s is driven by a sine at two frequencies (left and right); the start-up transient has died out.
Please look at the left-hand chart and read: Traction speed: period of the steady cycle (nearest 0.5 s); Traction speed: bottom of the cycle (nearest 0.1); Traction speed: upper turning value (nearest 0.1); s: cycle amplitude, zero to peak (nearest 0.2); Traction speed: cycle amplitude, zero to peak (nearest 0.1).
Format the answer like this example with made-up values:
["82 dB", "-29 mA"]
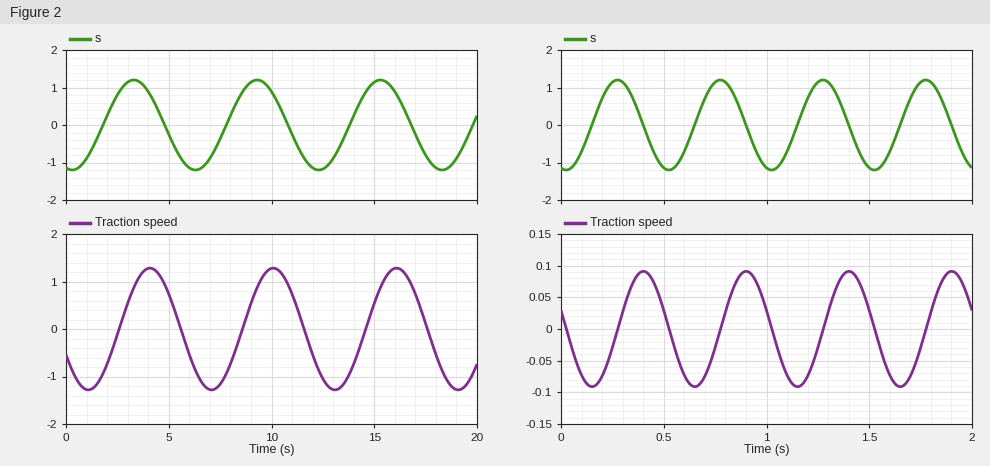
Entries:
["6.0 s", "-1.3", "1.3", "1.2", "1.3"]
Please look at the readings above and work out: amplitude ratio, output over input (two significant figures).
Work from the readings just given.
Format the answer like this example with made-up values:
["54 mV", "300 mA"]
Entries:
["1.1"]
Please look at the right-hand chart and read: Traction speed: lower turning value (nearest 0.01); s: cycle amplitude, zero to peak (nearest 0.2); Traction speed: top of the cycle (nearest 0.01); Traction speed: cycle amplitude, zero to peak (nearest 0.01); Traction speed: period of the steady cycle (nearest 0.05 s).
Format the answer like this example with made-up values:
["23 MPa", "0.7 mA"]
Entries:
["-0.09", "1.2", "0.09", "0.09", "0.50 s"]
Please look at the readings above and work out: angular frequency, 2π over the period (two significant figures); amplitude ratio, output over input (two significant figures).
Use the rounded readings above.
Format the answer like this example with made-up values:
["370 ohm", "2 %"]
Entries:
["13 rad/s", "0.075"]
